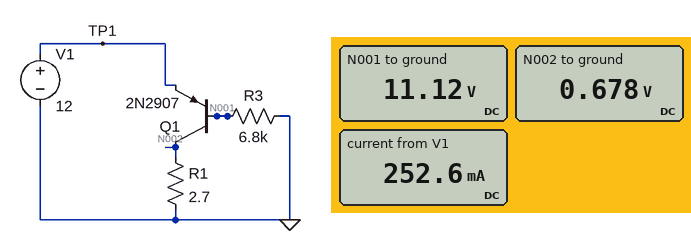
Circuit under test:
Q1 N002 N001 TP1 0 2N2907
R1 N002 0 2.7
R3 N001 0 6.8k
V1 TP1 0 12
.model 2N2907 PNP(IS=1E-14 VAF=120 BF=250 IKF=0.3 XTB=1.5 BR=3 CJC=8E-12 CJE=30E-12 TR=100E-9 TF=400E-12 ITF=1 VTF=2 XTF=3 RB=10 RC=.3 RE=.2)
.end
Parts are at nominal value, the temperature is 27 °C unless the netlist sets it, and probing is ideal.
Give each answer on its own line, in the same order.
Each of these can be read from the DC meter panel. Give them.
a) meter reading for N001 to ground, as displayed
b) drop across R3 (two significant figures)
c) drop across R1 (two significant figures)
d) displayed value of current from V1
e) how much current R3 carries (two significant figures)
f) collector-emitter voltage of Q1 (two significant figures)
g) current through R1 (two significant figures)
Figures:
11.12 V
11 V
680 mV
252.6 mA
1.6 mA
-11 V
250 mA
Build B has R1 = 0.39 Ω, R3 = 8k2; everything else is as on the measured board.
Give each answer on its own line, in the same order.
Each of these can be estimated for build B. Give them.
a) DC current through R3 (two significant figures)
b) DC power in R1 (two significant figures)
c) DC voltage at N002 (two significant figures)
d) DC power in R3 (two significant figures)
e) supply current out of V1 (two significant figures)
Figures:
1.4 mA
19 mW
86 mV
15 mW
220 mA
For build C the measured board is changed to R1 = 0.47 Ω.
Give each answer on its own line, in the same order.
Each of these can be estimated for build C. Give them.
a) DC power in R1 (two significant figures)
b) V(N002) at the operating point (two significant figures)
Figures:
30 mW
120 mV
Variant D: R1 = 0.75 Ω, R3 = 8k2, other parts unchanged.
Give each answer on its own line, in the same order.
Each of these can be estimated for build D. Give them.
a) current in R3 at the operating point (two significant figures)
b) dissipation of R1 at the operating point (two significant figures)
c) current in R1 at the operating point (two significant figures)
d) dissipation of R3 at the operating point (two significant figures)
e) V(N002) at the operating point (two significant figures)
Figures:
1.4 mA
37 mW
220 mA
15 mW
170 mV
